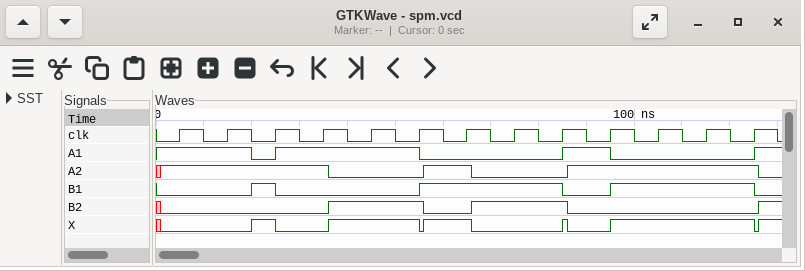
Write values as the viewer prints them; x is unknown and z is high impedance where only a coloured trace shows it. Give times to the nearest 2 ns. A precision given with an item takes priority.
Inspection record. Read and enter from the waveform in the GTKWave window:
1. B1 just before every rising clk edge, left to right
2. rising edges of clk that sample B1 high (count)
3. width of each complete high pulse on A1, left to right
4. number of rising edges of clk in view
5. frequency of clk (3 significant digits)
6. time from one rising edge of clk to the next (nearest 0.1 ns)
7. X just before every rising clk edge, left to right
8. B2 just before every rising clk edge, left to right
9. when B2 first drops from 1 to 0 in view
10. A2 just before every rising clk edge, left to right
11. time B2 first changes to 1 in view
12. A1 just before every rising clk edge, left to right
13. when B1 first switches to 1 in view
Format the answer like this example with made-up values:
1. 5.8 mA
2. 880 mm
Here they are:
1. 0 0 1 0 0 0 1 1 1 0 1 1 1
2. 7
3. 30 ns, 10 ns
4. 13
5. 100 MHz
6. 10 ns
7. 0 0 1 0 1 1 1 0 0 0 1 1 1
8. 0 0 0 0 1 1 0 1 1 0 0 0 0
9. 56 ns
10. 1 1 1 1 0 0 1 0 0 1 1 1 1
11. 36 ns
12. 1 1 0 1 1 1 0 0 0 1 0 0 0
13. 20 ns
